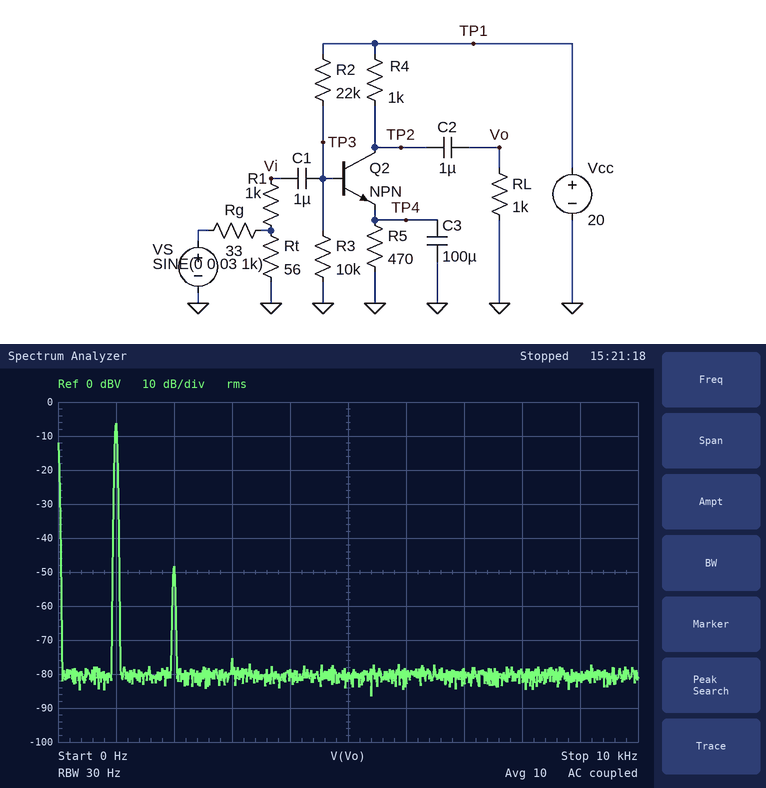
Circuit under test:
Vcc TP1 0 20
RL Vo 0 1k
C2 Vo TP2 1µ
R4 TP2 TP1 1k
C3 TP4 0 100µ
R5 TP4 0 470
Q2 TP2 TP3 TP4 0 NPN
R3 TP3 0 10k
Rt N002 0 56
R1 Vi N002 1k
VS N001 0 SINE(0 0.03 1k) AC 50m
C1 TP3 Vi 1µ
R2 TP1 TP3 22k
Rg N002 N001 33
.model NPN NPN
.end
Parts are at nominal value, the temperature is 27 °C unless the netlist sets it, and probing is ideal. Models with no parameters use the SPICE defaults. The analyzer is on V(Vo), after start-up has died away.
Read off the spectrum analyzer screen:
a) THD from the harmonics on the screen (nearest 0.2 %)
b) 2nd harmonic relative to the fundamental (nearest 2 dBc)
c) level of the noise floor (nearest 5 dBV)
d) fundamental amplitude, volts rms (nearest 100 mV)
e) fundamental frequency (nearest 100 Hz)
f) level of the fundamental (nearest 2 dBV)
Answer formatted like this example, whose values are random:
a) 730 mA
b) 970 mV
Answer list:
a) 0.8 %
b) -42 dBc
c) -80 dBV
d) 500 mV
e) 1.0 kHz
f) -6 dBV
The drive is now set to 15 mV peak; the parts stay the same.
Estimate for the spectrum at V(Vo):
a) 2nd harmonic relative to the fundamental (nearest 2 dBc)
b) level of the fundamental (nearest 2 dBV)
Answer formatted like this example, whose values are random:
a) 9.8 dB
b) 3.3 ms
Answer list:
a) -48 dBc
b) -12 dBV
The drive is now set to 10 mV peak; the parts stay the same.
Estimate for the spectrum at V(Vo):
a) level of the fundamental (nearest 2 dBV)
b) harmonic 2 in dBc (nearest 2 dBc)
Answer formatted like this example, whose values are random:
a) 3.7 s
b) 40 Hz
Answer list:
a) -16 dBV
b) -52 dBc
